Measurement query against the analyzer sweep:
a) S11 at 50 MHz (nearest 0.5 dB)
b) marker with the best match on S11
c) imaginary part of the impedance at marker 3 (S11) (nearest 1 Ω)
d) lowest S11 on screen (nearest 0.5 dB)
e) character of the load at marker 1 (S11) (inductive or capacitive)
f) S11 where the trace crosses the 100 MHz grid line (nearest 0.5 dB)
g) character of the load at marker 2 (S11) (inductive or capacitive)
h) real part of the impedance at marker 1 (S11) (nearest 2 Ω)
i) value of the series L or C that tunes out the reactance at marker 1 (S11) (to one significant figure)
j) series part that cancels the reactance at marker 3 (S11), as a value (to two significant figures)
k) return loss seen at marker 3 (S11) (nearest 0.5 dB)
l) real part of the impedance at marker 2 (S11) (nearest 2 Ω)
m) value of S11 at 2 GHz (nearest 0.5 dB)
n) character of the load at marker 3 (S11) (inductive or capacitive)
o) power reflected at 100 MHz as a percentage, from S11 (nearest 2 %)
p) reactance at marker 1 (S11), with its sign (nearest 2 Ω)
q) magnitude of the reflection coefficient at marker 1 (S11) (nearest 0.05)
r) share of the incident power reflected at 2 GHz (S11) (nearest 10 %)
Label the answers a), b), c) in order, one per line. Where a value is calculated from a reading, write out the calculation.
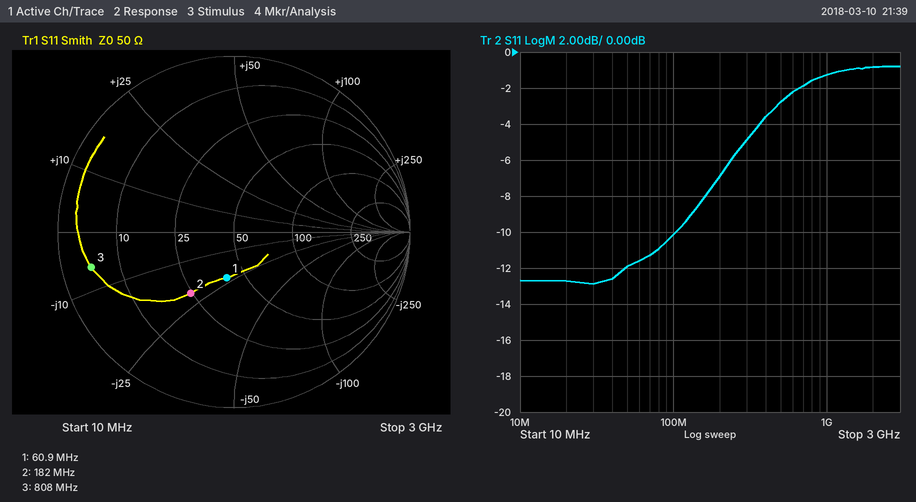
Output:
a) -12.0 dB
b) marker 1
c) -6 Ω
d) -13.0 dB
e) capacitive
f) -10.0 dB
g) capacitive
h) 40 Ω
i) L = 22 Ω/(2π × 60.9 MHz) ≈ 57.5 nH, so 60 nH to one significant figure
j) L = 6 Ω/(2π × 808 MHz) ≈ 1.2 nH
k) 1.5 dB
l) 24 Ω
m) -1.0 dB
n) capacitive
o) 10^(-10/10) ≈ 10 %
p) -22 Ω
q) 0.25
r) 10^(-1/10) ≈ 79.4 %, so 80 % to the nearest 10 %
